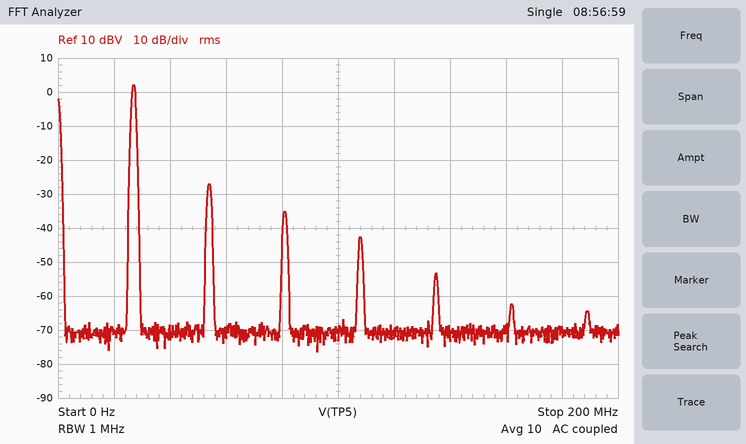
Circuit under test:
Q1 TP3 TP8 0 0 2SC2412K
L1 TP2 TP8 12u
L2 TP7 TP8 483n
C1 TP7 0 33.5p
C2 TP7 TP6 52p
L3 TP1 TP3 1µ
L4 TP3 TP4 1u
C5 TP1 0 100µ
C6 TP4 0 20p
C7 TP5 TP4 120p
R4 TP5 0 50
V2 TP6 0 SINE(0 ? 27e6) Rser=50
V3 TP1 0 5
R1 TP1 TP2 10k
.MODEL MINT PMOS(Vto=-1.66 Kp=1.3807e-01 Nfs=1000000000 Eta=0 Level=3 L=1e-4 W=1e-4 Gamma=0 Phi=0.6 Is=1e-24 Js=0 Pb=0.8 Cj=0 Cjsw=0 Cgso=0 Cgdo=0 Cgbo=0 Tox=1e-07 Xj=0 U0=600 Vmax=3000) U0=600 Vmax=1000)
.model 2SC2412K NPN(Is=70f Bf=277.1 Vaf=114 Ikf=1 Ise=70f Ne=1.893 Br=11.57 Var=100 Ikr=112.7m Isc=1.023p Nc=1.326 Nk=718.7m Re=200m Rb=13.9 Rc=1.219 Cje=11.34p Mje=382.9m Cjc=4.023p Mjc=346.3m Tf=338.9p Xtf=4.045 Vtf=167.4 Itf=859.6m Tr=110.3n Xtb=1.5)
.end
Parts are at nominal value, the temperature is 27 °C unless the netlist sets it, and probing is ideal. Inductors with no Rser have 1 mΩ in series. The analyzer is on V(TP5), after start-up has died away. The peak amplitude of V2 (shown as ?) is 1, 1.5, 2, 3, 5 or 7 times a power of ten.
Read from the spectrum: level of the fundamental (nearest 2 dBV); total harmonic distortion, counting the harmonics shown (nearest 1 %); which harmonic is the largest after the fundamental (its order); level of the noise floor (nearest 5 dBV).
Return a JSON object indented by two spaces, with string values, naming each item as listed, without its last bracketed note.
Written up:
{
  "level of the fundamental": "2 dBV",
  "total harmonic distortion, counting the harmonics shown": "4 %",
  "which harmonic is the largest after the fundamental": "2",
  "level of the noise floor": "-70 dBV"
}
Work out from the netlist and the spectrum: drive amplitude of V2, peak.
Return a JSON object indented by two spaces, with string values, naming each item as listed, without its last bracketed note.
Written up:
{
  "drive amplitude of V2, peak": "300 mV"
}
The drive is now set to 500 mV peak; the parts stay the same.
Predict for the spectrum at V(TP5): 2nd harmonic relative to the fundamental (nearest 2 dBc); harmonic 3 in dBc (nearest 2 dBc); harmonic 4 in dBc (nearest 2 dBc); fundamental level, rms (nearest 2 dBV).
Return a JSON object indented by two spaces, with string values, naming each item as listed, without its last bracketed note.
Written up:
{
  "2nd harmonic relative to the fundamental": "-16 dBc",
  "harmonic 3 in dBc": "-40 dBc",
  "harmonic 4 in dBc": "-32 dBc",
  "fundamental level, rms": "4 dBV"
}
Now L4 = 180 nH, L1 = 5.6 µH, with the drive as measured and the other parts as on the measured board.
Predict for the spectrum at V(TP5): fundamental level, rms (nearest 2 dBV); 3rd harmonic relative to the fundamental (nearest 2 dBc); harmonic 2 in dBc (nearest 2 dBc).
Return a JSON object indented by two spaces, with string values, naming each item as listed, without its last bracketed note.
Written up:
{
  "fundamental level, rms": "6 dBV",
  "3rd harmonic relative to the fundamental": "-56 dBc",
  "harmonic 2 in dBc": "-28 dBc"
}
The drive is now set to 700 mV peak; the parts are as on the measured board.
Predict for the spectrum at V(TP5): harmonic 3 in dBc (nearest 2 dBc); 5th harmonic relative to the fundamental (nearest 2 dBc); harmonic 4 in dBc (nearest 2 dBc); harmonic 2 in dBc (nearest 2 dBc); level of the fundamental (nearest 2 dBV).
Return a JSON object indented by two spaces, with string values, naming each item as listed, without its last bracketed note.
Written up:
{
  "harmonic 3 in dBc": "-32 dBc",
  "5th harmonic relative to the fundamental": "-32 dBc",
  "harmonic 4 in dBc": "-30 dBc",
  "harmonic 2 in dBc": "-16 dBc",
  "level of the fundamental": "4 dBV"
}
